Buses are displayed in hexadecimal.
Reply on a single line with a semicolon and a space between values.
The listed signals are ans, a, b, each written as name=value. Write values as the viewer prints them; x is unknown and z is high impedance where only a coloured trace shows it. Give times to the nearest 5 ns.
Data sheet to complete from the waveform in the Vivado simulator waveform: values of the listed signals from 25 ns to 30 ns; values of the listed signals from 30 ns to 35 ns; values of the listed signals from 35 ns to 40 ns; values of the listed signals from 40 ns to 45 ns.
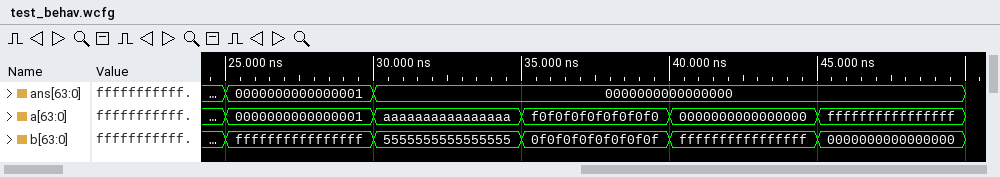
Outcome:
ans=0000000000000001, a=0000000000000001, b=ffffffffffffffff; ans=0000000000000000, a=aaaaaaaaaaaaaaaa, b=5555555555555555; ans=0000000000000000, a=f0f0f0f0f0f0f0f0, b=0f0f0f0f0f0f0f0f; ans=0000000000000000, a=0000000000000000, b=ffffffffffffffff
